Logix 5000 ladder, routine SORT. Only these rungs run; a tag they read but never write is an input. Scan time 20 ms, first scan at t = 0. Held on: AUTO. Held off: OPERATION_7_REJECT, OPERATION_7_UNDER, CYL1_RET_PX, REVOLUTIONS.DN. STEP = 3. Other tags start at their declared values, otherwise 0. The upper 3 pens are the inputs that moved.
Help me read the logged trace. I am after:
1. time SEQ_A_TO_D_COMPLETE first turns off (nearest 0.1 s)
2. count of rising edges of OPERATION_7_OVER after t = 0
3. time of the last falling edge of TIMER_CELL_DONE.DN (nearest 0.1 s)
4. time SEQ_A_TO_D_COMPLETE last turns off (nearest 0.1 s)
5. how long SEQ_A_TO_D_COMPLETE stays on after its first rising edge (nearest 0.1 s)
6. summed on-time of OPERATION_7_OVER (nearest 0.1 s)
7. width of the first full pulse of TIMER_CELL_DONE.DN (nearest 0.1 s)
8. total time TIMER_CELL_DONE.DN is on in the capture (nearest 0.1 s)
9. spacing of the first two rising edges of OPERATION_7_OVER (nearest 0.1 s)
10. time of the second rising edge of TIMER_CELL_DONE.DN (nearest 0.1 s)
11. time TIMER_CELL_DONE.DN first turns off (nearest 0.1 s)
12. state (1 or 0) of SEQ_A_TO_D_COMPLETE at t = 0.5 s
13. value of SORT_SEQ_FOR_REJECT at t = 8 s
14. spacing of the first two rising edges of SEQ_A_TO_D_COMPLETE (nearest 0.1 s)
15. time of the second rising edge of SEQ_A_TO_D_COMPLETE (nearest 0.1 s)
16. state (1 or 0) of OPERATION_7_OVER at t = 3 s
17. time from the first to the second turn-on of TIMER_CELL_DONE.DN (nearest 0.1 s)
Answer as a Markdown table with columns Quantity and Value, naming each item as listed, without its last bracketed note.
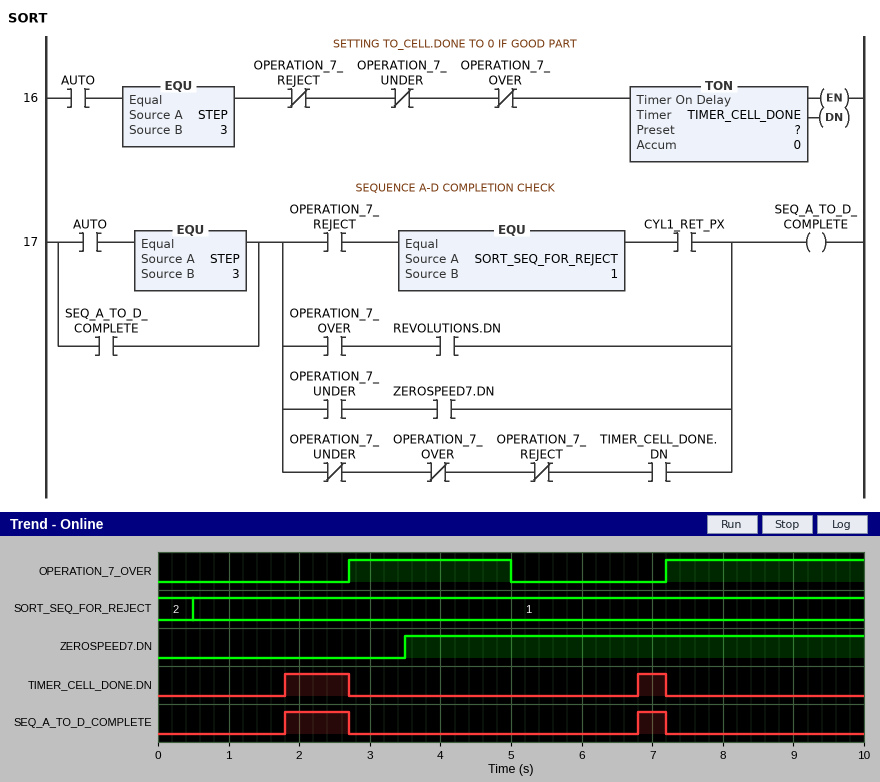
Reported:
| Quantity | Value |
|---|---|
| time SEQ_A_TO_D_COMPLETE first turns off | 2.7 s |
| count of rising edges of OPERATION_7_OVER after t = 0 | 2 |
| time of the last falling edge of TIMER_CELL_DONE.DN | 7.2 s |
| time SEQ_A_TO_D_COMPLETE last turns off | 7.2 s |
| how long SEQ_A_TO_D_COMPLETE stays on after its first rising edge | 0.9 s |
| summed on-time of OPERATION_7_OVER | 5.1 s |
| width of the first full pulse of TIMER_CELL_DONE.DN | 0.9 s |
| total time TIMER_CELL_DONE.DN is on in the capture | 1.3 s |
| spacing of the first two rising edges of OPERATION_7_OVER | 4.5 s |
| time of the second rising edge of TIMER_CELL_DONE.DN | 6.8 s |
| time TIMER_CELL_DONE.DN first turns off | 2.7 s |
| state (1 or 0) of SEQ_A_TO_D_COMPLETE at t = 0.5 s | 0 |
| value of SORT_SEQ_FOR_REJECT at t = 8 s | 1 |
| spacing of the first two rising edges of SEQ_A_TO_D_COMPLETE | 5.0 s |
| time of the second rising edge of SEQ_A_TO_D_COMPLETE | 6.8 s |
| state (1 or 0) of OPERATION_7_OVER at t = 3 s | 1 |
| time from the first to the second turn-on of TIMER_CELL_DONE.DN | 5.0 s |
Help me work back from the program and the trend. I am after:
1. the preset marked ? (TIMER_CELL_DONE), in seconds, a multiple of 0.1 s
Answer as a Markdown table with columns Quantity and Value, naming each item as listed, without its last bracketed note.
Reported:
| Quantity | Value |
|---|---|
| the preset marked ? (TIMER_CELL_DONE), in seconds, a multiple of 0.1 s | 1.8 s |
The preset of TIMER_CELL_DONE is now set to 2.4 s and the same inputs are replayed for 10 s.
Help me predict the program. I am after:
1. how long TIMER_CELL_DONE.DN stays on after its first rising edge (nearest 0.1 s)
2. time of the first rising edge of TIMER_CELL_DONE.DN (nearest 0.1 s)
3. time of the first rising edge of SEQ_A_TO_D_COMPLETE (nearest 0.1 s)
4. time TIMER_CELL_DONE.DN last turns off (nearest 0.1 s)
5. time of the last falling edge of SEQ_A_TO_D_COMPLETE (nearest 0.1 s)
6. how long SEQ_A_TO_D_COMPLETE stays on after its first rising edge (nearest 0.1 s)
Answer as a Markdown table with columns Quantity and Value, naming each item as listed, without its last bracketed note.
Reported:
| Quantity | Value |
|---|---|
| how long TIMER_CELL_DONE.DN stays on after its first rising edge | 0.3 s |
| time of the first rising edge of TIMER_CELL_DONE.DN | 2.4 s |
| time of the first rising edge of SEQ_A_TO_D_COMPLETE | 2.4 s |
| time TIMER_CELL_DONE.DN last turns off | 2.7 s |
| time of the last falling edge of SEQ_A_TO_D_COMPLETE | 2.7 s |
| how long SEQ_A_TO_D_COMPLETE stays on after its first rising edge | 0.3 s |
